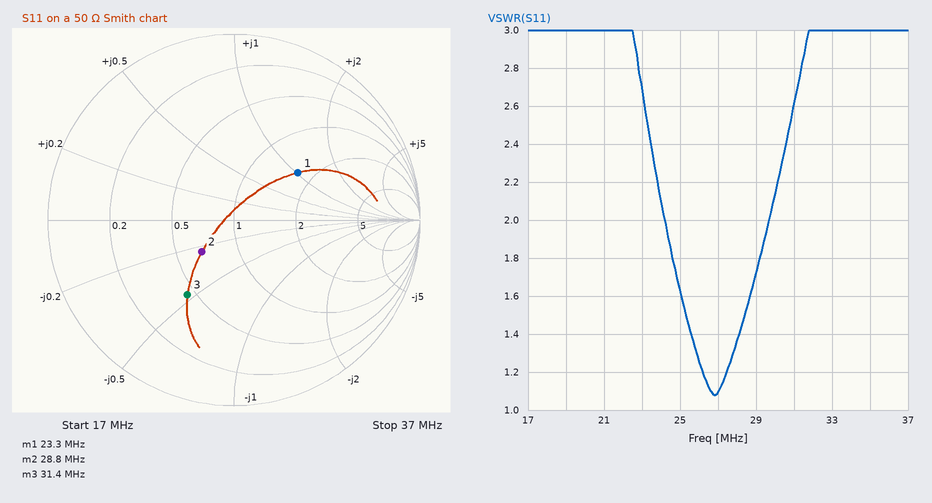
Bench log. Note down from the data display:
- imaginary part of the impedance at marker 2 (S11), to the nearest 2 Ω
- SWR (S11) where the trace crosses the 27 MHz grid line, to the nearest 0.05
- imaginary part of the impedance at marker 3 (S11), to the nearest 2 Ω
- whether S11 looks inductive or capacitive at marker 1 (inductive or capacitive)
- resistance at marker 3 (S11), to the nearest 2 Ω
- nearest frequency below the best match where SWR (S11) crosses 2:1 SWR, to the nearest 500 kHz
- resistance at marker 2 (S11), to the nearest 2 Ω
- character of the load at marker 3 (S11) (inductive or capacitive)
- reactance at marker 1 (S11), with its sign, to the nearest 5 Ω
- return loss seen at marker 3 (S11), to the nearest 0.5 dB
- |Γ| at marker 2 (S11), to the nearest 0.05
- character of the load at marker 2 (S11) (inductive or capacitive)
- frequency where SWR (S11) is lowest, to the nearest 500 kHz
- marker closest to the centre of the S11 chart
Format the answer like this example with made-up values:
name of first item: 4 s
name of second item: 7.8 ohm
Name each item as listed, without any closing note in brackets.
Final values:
imaginary part of the impedance at marker 2 (S11), to the nearest 2 Ω: -12 Ω
SWR (S11) where the trace crosses the 27 MHz grid line, to the nearest 0.05: 1.10
imaginary part of the impedance at marker 3 (S11), to the nearest 2 Ω: -24 Ω
whether S11 looks inductive or capacitive at marker 1: inductive
resistance at marker 3 (S11), to the nearest 2 Ω: 22 Ω
nearest frequency below the best match where SWR (S11) crosses 2:1 SWR, to the nearest 500 kHz: 24.0 MHz
resistance at marker 2 (S11), to the nearest 2 Ω: 34 Ω
character of the load at marker 3 (S11): capacitive
reactance at marker 1 (S11), with its sign, to the nearest 5 Ω: +50 Ω
return loss seen at marker 3 (S11), to the nearest 0.5 dB: 6.5 dB
|Γ| at marker 2 (S11), to the nearest 0.05: 0.25
character of the load at marker 2 (S11): capacitive
frequency where SWR (S11) is lowest, to the nearest 500 kHz: 27.0 MHz
marker closest to the centre of the S11 chart: marker 2
